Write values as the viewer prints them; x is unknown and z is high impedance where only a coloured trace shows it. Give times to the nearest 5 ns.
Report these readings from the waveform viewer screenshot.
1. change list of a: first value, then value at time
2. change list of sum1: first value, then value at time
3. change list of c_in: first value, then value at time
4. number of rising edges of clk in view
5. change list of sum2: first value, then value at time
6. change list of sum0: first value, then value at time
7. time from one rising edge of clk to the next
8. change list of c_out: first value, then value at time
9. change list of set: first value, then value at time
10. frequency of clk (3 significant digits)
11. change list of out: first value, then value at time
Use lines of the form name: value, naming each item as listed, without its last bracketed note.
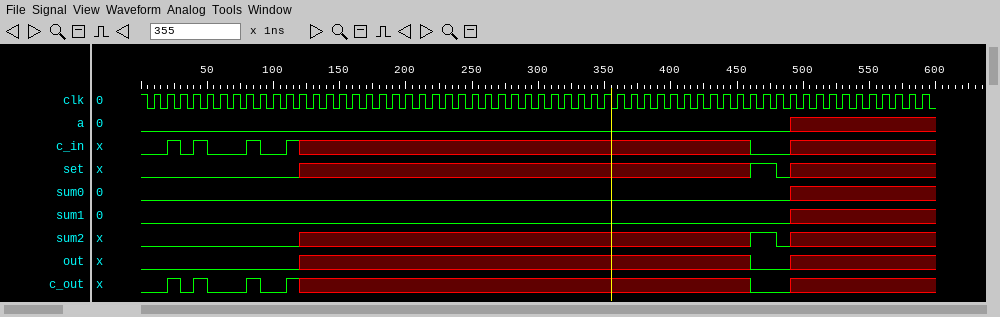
change list of a: first value, then value at time: 0, x at 490 ns
change list of sum1: first value, then value at time: 0, x at 490 ns
change list of c_in: first value, then value at time: 0, 1 at 20 ns, 0 at 30 ns, 1 at 40 ns, 0 at 50 ns, 1 at 80 ns, 0 at 90 ns, 1 at 110 ns, x at 120 ns, 0 at 460 ns, x at 490 ns
number of rising edges of clk in view: 59
change list of sum2: first value, then value at time: 0, x at 120 ns, 1 at 460 ns, 0 at 480 ns, x at 490 ns
change list of sum0: first value, then value at time: 0, x at 490 ns
time from one rising edge of clk to the next: 10 ns
change list of c_out: first value, then value at time: 0, 1 at 20 ns, 0 at 30 ns, 1 at 40 ns, 0 at 50 ns, 1 at 80 ns, 0 at 90 ns, 1 at 110 ns, x at 120 ns, 0 at 460 ns, x at 490 ns
change list of set: first value, then value at time: 0, x at 120 ns, 1 at 460 ns, 0 at 480 ns, x at 490 ns
frequency of clk: 100 MHz
change list of out: first value, then value at time: 0, x at 120 ns, 0 at 460 ns, x at 490 ns
